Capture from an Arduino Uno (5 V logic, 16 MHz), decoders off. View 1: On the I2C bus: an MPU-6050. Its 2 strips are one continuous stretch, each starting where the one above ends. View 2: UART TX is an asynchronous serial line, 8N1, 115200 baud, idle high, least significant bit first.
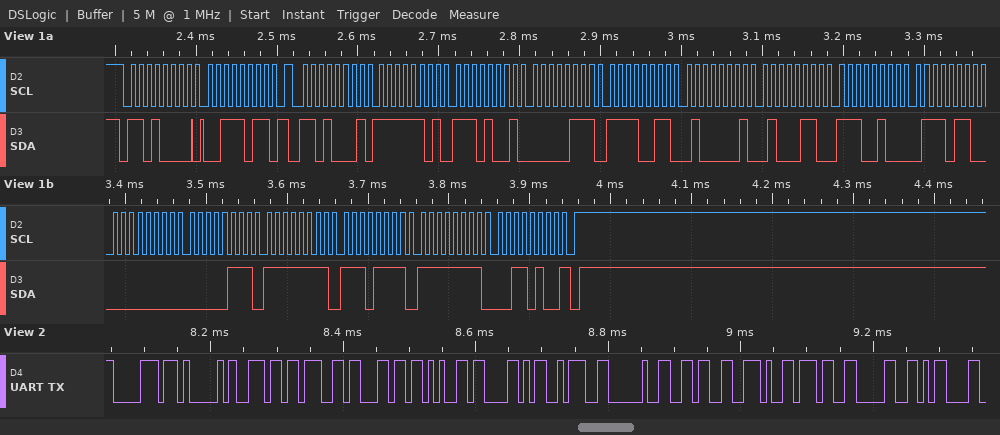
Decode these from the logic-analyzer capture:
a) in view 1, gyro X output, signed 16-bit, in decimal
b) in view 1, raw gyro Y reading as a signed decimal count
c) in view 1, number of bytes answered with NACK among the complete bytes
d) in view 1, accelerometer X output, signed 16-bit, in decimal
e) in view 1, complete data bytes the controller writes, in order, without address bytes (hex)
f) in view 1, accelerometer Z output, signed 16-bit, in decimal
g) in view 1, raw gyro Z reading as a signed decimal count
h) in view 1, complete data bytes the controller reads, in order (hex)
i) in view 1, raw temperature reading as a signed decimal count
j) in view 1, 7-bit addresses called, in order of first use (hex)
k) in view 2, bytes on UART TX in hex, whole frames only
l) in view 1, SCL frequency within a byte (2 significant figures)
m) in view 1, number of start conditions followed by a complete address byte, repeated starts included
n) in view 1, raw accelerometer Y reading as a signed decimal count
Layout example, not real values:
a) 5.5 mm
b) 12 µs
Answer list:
a) 7
b) -17
c) 1
d) -535
e) 3B
f) 16710
g) -204
h) FD E9 07 F3 41 46 E4 76 00 07 FF EF FF 34
i) -7050
j) 0x68
k) 0x70 0x41 0x6E 0x67 0x6C 0x65 0x58 0x3A 0x20 0x36 0x2E 0x37 0x30 0x0D
l) 100 kHz
m) 2
n) 2035
